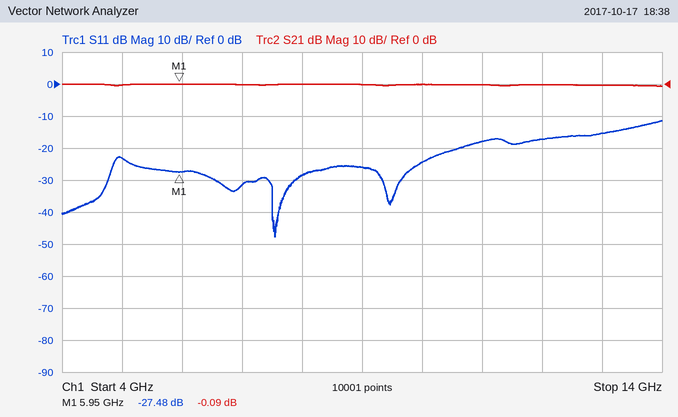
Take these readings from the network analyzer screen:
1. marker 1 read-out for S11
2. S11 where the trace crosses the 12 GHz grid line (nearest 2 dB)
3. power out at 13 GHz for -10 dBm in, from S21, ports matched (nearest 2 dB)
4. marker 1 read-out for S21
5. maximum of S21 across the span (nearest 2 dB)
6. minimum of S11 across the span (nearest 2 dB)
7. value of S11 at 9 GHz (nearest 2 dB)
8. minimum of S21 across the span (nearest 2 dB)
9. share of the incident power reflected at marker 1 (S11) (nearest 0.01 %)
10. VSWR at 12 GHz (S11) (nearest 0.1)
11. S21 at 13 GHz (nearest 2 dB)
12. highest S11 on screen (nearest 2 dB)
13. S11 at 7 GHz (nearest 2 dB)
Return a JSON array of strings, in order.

["-27.48 dB", "-18 dB", "-10 dBm", "-0.09 dB", "0 dB", "-48 dB", "-26 dB", "0 dB", "0.18 %", "1.3", "0 dB", "-12 dB", "-32 dB"]
